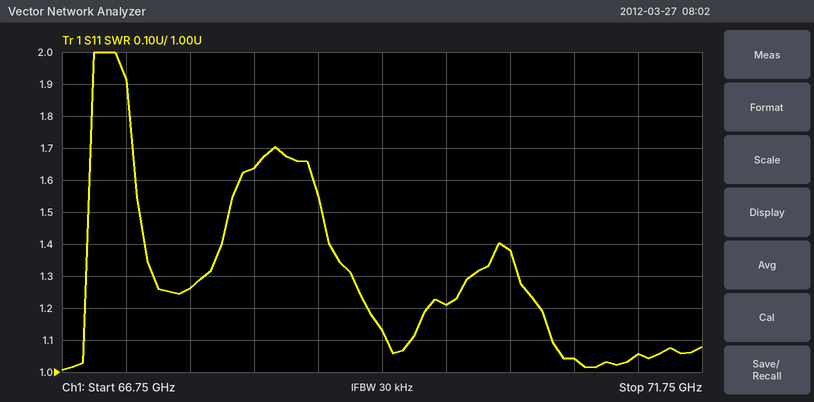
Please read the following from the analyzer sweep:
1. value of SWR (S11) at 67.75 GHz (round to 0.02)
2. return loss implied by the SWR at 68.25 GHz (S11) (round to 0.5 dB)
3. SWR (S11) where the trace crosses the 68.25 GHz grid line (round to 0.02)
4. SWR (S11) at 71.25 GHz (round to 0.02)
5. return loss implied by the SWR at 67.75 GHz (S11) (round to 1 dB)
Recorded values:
1.26
12.5 dB
1.64
1.06
19 dB
